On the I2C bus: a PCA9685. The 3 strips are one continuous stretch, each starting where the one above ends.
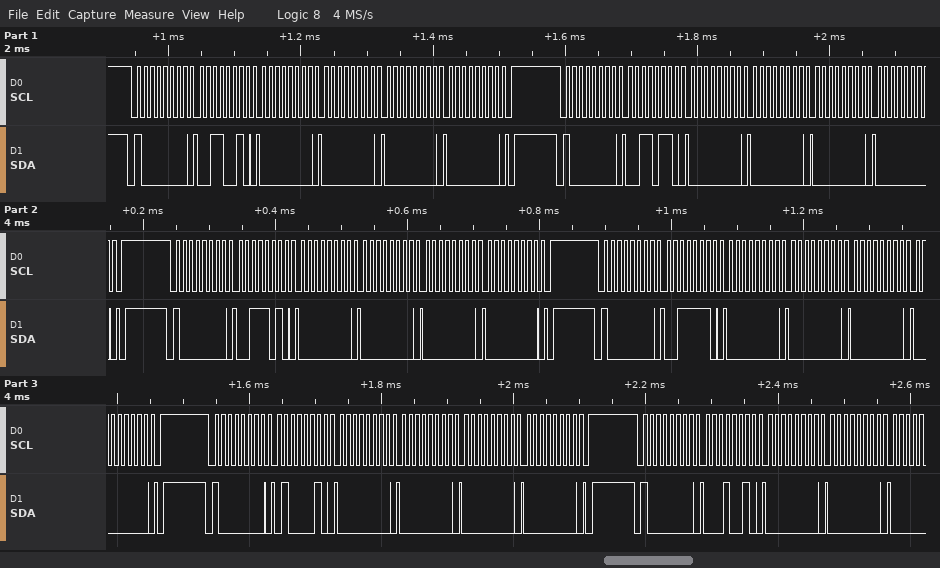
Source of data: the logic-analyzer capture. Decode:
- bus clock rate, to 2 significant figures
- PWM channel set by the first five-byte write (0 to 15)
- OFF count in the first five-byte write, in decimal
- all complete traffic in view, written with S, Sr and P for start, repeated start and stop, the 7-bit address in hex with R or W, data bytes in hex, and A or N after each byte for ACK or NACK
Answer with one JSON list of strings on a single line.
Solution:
["100 kHz", "11", "0", "S 40W A 32 A 00 A 00 A 00 A 00 A P S 40W A 36 A 00 A 00 A 00 A 00 A P S 40W A 3A A 00 A 00 A 00 A 00 A P S 40W A 3E A 00 A 00 A 00 A 00 A P S 40W A 42 A 00 A 00 A 00 A 00 A P S 40W A 12 A 00 A 00 A"]
